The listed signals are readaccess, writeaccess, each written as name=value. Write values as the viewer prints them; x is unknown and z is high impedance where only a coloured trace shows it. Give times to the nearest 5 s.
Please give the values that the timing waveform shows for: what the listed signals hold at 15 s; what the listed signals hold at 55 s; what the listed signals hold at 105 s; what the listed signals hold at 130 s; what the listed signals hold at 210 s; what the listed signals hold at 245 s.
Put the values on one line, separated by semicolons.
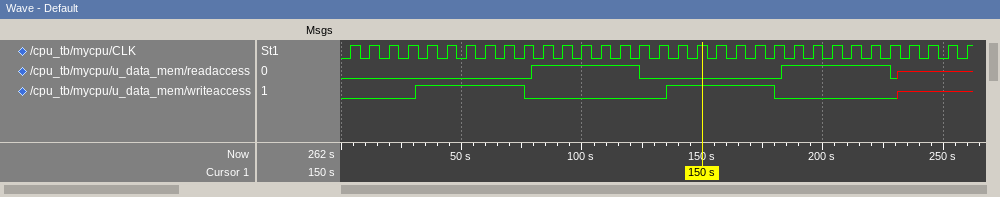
readaccess=0, writeaccess=0; readaccess=0, writeaccess=1; readaccess=1, writeaccess=0; readaccess=0, writeaccess=0; readaccess=1, writeaccess=0; readaccess=x, writeaccess=x
